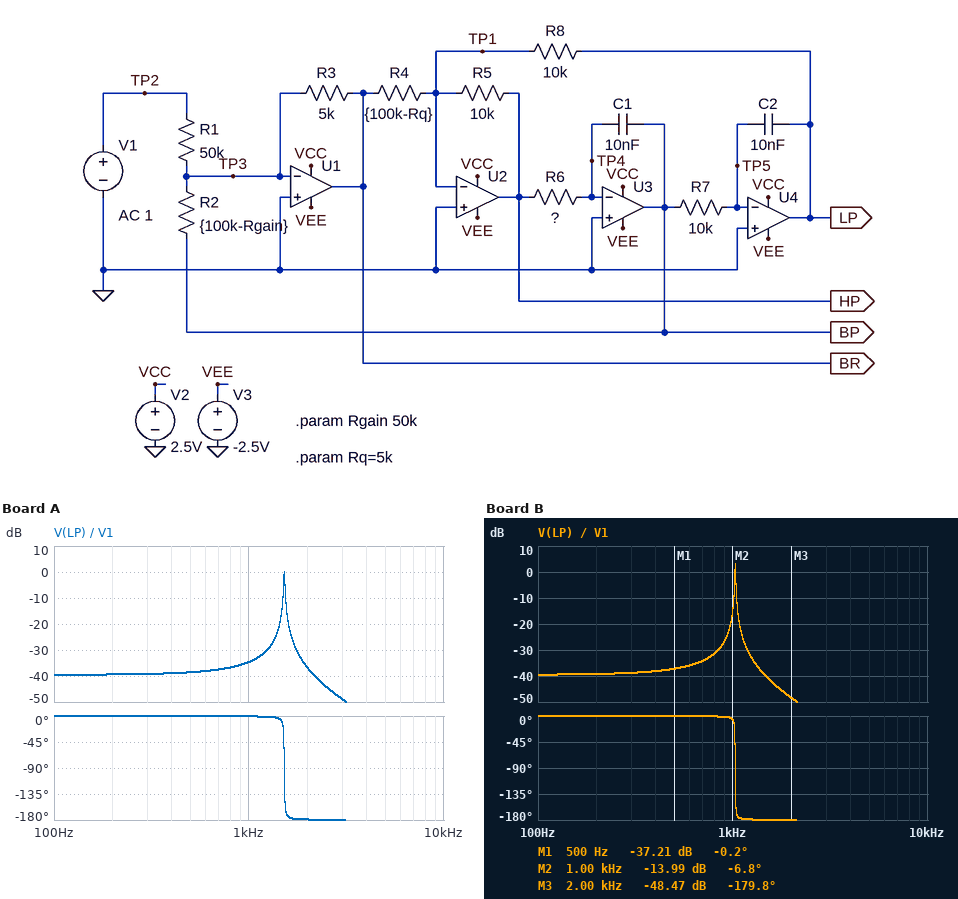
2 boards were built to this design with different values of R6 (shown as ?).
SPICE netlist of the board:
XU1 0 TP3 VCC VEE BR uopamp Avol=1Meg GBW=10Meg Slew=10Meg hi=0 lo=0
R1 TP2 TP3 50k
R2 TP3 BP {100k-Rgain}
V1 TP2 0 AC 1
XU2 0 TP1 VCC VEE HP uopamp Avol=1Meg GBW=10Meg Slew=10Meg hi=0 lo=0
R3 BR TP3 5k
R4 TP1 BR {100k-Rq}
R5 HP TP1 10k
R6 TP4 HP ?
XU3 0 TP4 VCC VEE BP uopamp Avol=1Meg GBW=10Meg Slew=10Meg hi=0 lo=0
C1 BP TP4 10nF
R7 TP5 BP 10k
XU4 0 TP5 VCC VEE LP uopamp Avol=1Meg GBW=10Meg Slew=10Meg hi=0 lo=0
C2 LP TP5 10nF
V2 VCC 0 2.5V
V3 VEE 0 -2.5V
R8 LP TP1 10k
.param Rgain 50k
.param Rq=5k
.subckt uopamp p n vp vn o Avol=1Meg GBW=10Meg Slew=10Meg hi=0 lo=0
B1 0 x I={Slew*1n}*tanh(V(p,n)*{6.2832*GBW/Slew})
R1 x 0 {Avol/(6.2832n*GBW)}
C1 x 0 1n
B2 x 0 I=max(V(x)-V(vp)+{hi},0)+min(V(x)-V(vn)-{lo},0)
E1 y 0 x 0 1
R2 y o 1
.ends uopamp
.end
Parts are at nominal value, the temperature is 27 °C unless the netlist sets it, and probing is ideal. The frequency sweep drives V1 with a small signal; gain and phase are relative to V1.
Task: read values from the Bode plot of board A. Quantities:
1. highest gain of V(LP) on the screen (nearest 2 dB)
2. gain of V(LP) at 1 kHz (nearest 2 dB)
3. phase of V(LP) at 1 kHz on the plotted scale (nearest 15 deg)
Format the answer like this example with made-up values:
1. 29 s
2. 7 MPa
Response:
1. 0 dB
2. -34 dB
3. 0 deg
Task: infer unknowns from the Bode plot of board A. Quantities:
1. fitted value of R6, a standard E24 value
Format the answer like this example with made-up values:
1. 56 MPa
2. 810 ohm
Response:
1. 11 kΩ
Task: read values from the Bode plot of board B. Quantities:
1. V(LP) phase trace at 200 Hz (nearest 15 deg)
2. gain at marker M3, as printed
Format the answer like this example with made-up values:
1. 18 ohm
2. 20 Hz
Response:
1. 0 deg
2. -48.47 dB
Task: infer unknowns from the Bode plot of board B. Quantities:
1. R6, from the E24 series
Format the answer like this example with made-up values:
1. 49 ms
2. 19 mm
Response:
1. 24 kΩ
